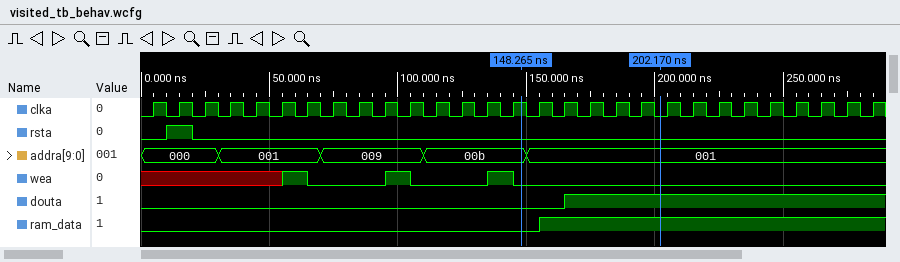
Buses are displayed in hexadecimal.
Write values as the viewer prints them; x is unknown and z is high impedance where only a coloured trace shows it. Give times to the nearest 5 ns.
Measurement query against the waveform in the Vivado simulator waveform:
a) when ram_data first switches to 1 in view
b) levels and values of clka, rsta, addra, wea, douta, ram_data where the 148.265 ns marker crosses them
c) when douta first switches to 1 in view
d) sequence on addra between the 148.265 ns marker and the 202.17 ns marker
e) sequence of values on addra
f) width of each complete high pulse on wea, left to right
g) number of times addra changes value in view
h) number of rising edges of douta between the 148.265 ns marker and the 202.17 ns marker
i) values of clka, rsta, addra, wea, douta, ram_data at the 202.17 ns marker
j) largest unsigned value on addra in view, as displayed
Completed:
155 ns
clka=1, rsta=0, addra=00b, wea=0, douta=0, ram_data=0
165 ns
00b, 001
000, 001, 009, 00b, 001
10 ns, 10 ns
4
1
clka=0, rsta=0, addra=001, wea=0, douta=1, ram_data=1
00b
